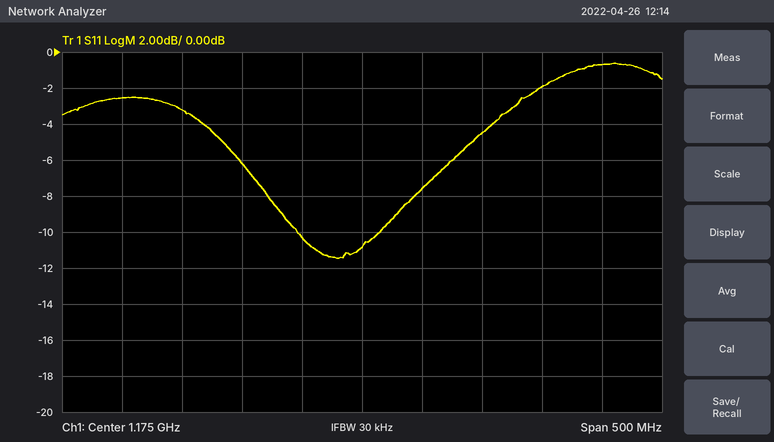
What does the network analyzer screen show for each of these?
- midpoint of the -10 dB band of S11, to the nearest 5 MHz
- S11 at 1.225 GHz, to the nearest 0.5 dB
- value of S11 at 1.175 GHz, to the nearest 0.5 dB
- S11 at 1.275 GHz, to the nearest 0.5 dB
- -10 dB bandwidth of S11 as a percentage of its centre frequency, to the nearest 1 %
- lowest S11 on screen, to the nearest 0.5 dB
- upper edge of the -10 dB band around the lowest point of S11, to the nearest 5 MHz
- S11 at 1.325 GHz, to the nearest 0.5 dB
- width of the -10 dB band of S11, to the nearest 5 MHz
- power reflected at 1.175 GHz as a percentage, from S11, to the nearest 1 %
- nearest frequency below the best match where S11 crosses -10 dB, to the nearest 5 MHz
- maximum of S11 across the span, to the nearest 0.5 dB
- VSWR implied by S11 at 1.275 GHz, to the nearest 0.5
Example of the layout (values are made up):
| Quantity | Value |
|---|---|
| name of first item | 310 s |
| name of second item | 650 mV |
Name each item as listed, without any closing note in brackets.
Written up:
| Quantity | Value |
|---|---|
| midpoint of the -10 dB band of S11, to the nearest 5 MHz | 1.155 GHz |
| S11 at 1.225 GHz, to the nearest 0.5 dB | -7.5 dB |
| value of S11 at 1.175 GHz, to the nearest 0.5 dB | -11.0 dB |
| S11 at 1.275 GHz, to the nearest 0.5 dB | -4.5 dB |
| -10 dB bandwidth of S11 as a percentage of its centre frequency, to the nearest 1 % | 6 % |
| lowest S11 on screen, to the nearest 0.5 dB | -11.5 dB |
| upper edge of the -10 dB band around the lowest point of S11, to the nearest 5 MHz | 1.190 GHz |
| S11 at 1.325 GHz, to the nearest 0.5 dB | -2.0 dB |
| width of the -10 dB band of S11, to the nearest 5 MHz | 70 MHz |
| power reflected at 1.175 GHz as a percentage, from S11, to the nearest 1 % | 8 % |
| nearest frequency below the best match where S11 crosses -10 dB, to the nearest 5 MHz | 1.120 GHz |
| maximum of S11 across the span, to the nearest 0.5 dB | -0.5 dB |
| VSWR implied by S11 at 1.275 GHz, to the nearest 0.5 | 4.0 |
